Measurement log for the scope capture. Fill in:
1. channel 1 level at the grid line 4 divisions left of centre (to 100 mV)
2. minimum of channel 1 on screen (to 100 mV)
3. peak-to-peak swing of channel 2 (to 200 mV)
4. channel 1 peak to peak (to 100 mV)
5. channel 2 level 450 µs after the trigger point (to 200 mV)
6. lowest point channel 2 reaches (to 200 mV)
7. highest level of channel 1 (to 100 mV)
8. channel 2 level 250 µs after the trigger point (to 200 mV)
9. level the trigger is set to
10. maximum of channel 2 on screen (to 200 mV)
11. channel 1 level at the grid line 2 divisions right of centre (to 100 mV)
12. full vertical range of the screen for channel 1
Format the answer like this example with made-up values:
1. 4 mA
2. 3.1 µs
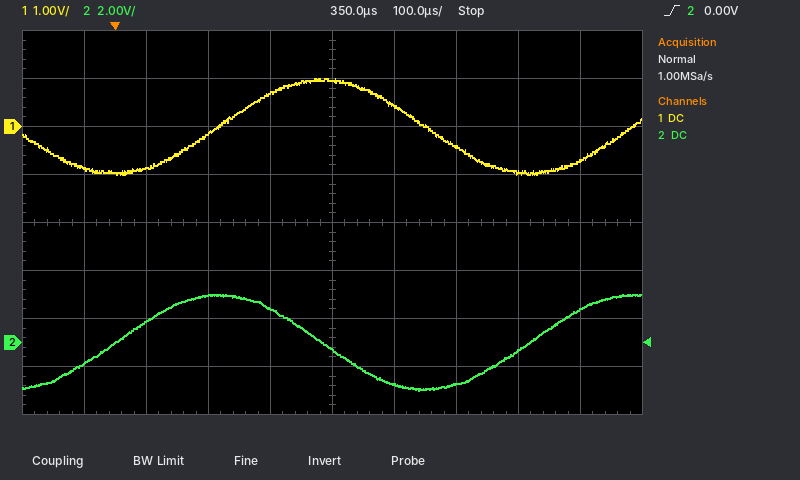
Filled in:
1. -900 mV
2. -1.0 V
3. 4.0 V
4. 2.0 V
5. -1.8 V
6. -2.0 V
7. 1.0 V
8. 1.4 V
9. 0.00 V
10. 2.0 V
11. -400 mV
12. 8 V
